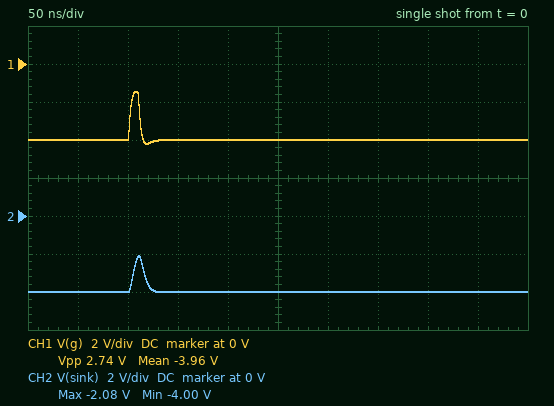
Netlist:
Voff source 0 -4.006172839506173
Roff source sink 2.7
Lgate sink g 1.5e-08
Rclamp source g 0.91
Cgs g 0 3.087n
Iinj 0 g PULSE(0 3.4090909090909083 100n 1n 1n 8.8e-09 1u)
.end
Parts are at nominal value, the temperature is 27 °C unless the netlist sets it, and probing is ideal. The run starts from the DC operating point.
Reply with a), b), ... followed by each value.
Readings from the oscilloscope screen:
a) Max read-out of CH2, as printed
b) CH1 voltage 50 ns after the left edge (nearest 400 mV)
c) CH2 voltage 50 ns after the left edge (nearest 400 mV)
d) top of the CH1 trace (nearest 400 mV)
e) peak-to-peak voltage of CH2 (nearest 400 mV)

a) -2.08 V
b) -4.0 V
c) -4.0 V
d) -1.6 V
e) 2.0 V
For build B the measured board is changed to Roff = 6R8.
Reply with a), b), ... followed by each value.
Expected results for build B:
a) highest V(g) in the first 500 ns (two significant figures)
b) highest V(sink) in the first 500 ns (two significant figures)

a) -1.3 V
b) -1.4 V
